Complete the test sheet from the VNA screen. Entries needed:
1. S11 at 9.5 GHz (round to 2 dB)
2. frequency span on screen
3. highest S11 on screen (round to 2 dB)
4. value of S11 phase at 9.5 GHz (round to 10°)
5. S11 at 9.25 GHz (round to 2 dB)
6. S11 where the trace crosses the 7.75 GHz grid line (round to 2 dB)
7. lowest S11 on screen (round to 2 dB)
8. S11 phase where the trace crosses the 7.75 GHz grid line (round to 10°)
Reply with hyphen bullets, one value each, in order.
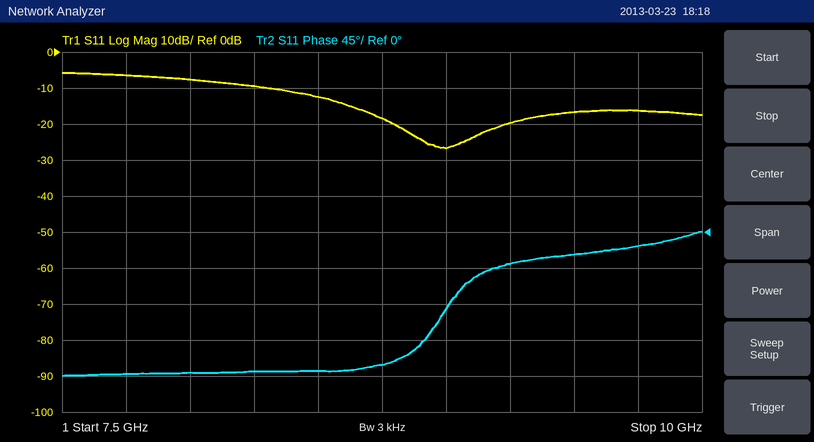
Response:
- -16 dB
- 2.5 GHz
- -6 dB
- -30°
- -20 dB
- -6 dB
- -26 dB
- -180°
